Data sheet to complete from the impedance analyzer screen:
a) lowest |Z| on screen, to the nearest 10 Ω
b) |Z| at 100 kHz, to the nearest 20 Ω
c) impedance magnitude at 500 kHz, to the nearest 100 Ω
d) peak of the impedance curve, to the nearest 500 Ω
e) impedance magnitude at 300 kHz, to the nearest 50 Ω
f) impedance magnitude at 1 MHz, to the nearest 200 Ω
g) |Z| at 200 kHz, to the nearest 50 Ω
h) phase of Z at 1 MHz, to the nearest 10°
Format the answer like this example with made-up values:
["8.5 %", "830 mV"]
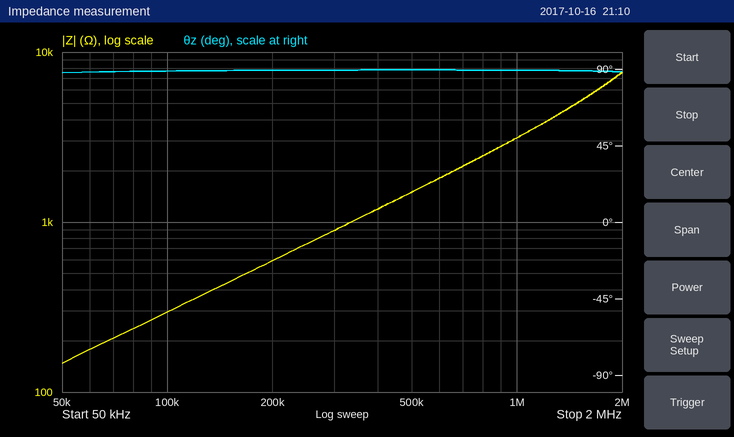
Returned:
["150 Ω", "300 Ω", "1.5 kΩ", "7.5 kΩ", "900 Ω", "3.2 kΩ", "600 Ω", "90°"]
